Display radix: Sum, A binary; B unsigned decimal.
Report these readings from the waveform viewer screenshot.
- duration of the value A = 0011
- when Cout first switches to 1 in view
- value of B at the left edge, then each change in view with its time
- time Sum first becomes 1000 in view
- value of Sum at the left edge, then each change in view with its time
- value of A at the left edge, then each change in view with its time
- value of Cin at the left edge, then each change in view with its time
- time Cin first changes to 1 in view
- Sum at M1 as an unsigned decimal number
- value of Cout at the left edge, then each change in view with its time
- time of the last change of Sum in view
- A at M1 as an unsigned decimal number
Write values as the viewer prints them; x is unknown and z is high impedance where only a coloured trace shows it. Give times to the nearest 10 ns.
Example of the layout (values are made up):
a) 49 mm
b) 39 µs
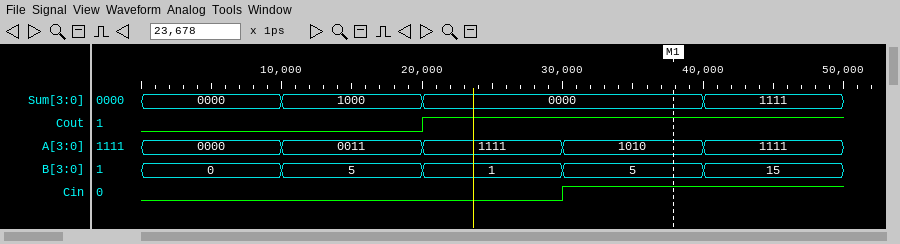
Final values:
a) 10 ns
b) 20 ns
c) 0, 5 at 10 ns, 1 at 20 ns, 5 at 30 ns, 15 at 40 ns
d) 10 ns
e) 0000, 1000 at 10 ns, 0000 at 20 ns, 1111 at 40 ns
f) 0000, 0011 at 10 ns, 1111 at 20 ns, 1010 at 30 ns, 1111 at 40 ns
g) 0, 1 at 30 ns
h) 30 ns
i) 0
j) 0, 1 at 20 ns
k) 40 ns
l) 10
